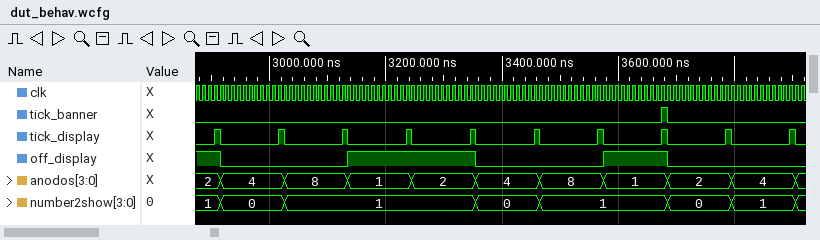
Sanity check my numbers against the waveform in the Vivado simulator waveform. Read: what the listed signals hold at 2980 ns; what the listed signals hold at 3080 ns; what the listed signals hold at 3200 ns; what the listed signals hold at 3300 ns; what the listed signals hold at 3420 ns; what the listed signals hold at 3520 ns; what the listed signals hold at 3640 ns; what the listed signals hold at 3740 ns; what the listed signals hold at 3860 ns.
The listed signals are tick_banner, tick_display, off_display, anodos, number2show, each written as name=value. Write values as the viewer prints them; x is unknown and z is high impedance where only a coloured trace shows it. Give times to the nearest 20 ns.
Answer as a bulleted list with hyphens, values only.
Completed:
- tick_banner=0, tick_display=0, off_display=0, anodos=4, number2show=0
- tick_banner=0, tick_display=0, off_display=0, anodos=8, number2show=1
- tick_banner=0, tick_display=0, off_display=1, anodos=1, number2show=1
- tick_banner=0, tick_display=0, off_display=1, anodos=2, number2show=1
- tick_banner=0, tick_display=0, off_display=0, anodos=4, number2show=0
- tick_banner=0, tick_display=0, off_display=0, anodos=8, number2show=1
- tick_banner=0, tick_display=0, off_display=1, anodos=1, number2show=1
- tick_banner=0, tick_display=0, off_display=0, anodos=2, number2show=0
- tick_banner=0, tick_display=0, off_display=0, anodos=4, number2show=1
